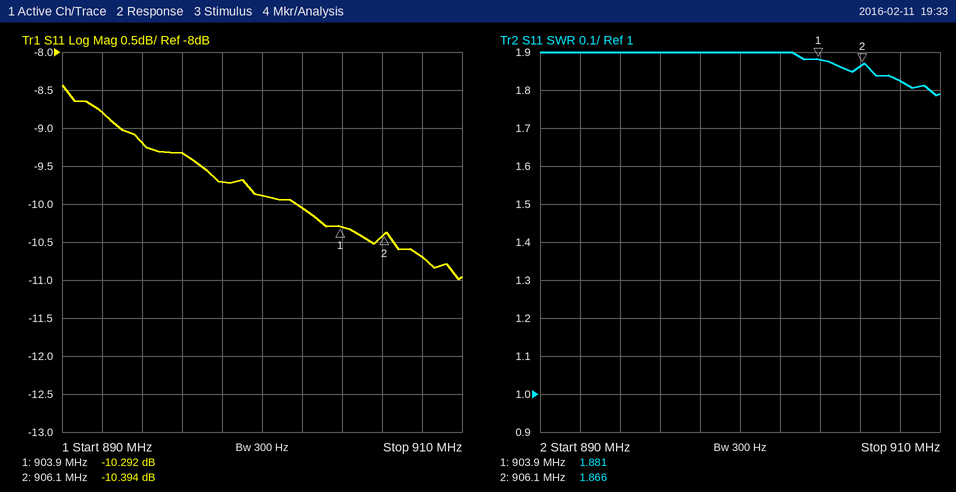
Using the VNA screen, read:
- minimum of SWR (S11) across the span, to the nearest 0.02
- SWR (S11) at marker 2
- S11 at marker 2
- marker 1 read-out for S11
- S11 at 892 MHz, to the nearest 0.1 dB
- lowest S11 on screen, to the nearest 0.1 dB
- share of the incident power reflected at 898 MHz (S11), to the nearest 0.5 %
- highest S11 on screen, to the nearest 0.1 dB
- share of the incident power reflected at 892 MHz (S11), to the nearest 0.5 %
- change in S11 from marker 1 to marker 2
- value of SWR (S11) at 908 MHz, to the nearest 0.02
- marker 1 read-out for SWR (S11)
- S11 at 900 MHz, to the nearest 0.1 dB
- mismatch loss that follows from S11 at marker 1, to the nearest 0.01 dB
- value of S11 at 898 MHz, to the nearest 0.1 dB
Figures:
1.78
1.866
-10.394 dB
-10.292 dB
-8.8 dB
-11.0 dB
10.5 %
-8.4 dB
13.0 %
-0.102 dB
1.82
1.881
-9.9 dB
0.43 dB
-9.7 dB
